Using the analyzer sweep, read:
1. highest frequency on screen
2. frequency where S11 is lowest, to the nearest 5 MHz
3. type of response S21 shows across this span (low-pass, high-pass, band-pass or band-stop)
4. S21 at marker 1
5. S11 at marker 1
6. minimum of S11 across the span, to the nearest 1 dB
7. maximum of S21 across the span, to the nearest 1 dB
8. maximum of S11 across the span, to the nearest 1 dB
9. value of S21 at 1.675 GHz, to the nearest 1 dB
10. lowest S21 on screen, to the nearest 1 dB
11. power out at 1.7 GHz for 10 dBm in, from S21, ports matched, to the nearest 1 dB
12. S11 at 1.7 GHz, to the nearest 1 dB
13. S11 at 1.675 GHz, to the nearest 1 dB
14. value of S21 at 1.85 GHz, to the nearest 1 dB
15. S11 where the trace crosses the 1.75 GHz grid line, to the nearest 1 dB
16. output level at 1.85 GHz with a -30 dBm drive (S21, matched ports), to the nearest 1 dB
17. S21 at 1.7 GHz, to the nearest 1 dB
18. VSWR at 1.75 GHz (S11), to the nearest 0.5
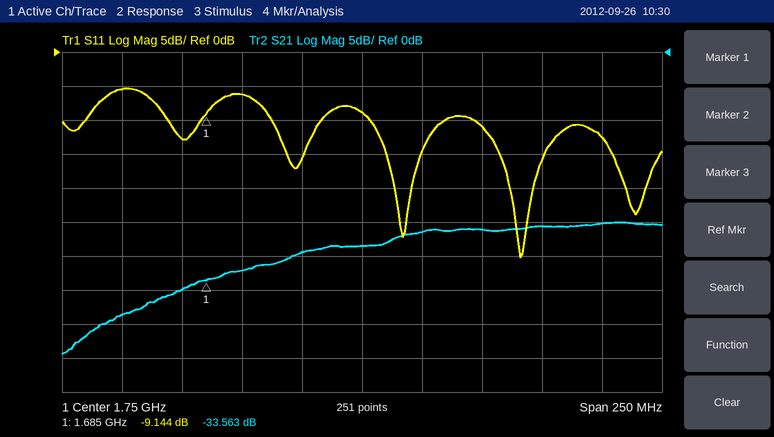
1.875 GHz
1.815 GHz
high-pass
-33.563 dB
-9.144 dB
-30 dB
-25 dB
-5 dB
-35 dB
-44 dB
-22 dBm
-6 dB
-13 dB
-25 dB
-9 dB
-55 dBm
-32 dB
2.0
